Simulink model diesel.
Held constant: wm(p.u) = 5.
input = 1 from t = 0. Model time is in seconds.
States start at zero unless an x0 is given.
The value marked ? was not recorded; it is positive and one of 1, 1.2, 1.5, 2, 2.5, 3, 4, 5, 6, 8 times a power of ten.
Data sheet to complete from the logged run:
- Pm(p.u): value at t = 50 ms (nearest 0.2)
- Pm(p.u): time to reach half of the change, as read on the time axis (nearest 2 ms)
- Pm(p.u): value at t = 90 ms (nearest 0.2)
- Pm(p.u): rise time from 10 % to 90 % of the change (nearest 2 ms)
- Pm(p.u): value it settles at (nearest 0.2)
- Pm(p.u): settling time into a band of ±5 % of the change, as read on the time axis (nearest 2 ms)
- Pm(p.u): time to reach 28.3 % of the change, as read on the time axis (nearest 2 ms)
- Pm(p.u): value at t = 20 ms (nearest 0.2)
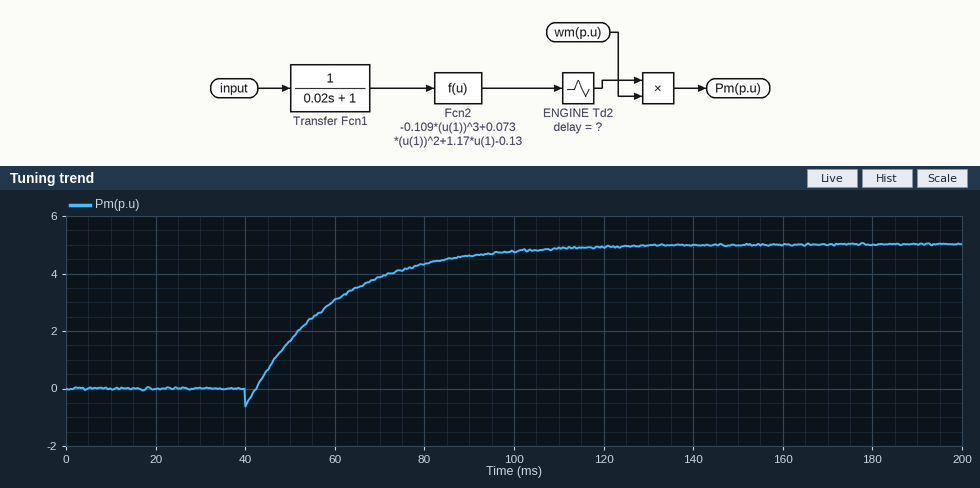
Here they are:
1.6
56 ms
4.6
42 ms
5.0
100 ms
48 ms
0.0
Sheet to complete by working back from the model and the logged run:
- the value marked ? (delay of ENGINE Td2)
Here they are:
0.04
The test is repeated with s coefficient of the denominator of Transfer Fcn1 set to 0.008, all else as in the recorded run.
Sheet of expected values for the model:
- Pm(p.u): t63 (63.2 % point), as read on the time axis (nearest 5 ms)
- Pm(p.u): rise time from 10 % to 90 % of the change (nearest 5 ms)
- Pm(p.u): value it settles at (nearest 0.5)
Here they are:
50 ms
15 ms
5.0
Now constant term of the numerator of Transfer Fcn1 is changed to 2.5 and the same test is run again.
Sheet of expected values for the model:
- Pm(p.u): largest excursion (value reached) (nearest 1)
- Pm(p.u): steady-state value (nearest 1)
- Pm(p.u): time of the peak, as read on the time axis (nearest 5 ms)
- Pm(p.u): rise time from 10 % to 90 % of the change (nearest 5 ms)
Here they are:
8
8
80 ms
15 ms
